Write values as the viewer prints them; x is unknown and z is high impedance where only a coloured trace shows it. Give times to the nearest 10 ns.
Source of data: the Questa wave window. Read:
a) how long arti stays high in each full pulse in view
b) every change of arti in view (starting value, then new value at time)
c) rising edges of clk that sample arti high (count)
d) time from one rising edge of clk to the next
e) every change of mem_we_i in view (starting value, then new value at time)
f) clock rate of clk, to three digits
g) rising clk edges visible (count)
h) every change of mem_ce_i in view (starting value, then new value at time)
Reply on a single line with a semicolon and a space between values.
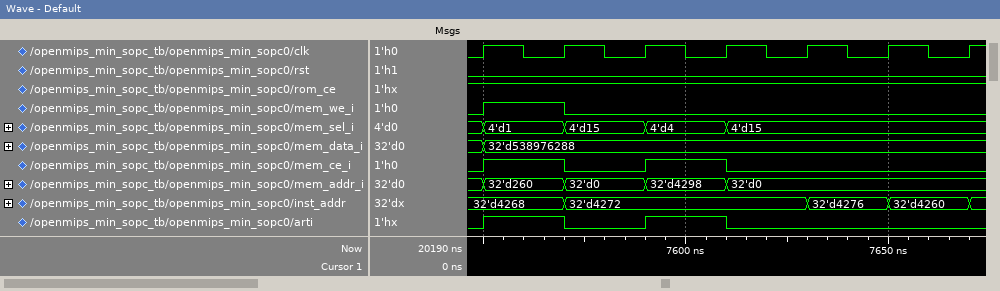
20 ns, 20 ns; 0, 1 at 7550 ns, 0 at 7570 ns, 1 at 7590 ns, 0 at 7610 ns; 2; 20 ns; 0, 1 at 7550 ns, 0 at 7570 ns; 50.0 MHz; 7; 0, 1 at 7550 ns, 0 at 7570 ns, 1 at 7590 ns, 0 at 7610 ns
